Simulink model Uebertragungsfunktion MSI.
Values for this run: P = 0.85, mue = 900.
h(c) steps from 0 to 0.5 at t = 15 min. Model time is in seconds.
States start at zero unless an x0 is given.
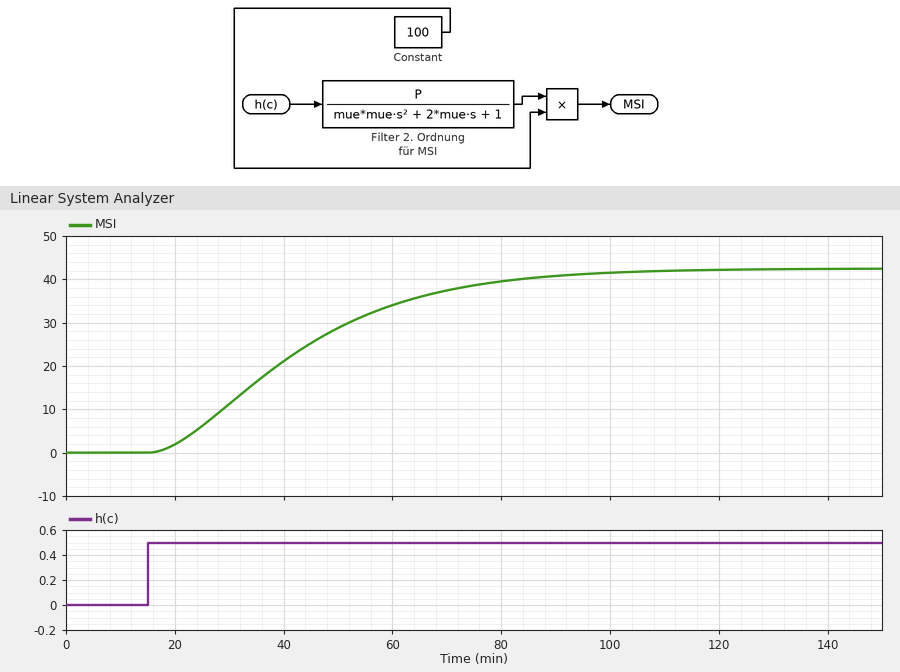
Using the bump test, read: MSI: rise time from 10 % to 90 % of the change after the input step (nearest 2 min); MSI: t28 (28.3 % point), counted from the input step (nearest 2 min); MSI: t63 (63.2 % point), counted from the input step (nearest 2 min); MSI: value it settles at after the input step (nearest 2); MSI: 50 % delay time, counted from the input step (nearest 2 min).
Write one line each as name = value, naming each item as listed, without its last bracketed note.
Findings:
MSI: rise time from 10 % to 90 % of the change after the input step = 50 min
MSI: t28 (28.3 % point), counted from the input step = 16 min
MSI: t63 (63.2 % point), counted from the input step = 32 min
MSI: value it settles at after the input step = 42
MSI: 50 % delay time, counted from the input step = 26 min
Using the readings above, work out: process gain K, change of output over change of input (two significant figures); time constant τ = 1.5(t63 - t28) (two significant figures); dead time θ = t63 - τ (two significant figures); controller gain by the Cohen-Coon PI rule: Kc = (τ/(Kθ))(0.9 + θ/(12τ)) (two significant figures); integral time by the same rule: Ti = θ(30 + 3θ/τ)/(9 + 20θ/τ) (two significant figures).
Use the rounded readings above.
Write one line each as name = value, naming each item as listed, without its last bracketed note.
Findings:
process gain K, change of output over change of input = 84
time constant τ = 1.5(t63 - t28) = 24 min
dead time θ = t63 - τ = 8.0 min
controller gain by the Cohen-Coon PI rule: Kc = (τ/(Kθ))(0.9 + θ/(12τ)) = 0.033
integral time by the same rule: Ti = θ(30 + 3θ/τ)/(9 + 20θ/τ) = 16 min
